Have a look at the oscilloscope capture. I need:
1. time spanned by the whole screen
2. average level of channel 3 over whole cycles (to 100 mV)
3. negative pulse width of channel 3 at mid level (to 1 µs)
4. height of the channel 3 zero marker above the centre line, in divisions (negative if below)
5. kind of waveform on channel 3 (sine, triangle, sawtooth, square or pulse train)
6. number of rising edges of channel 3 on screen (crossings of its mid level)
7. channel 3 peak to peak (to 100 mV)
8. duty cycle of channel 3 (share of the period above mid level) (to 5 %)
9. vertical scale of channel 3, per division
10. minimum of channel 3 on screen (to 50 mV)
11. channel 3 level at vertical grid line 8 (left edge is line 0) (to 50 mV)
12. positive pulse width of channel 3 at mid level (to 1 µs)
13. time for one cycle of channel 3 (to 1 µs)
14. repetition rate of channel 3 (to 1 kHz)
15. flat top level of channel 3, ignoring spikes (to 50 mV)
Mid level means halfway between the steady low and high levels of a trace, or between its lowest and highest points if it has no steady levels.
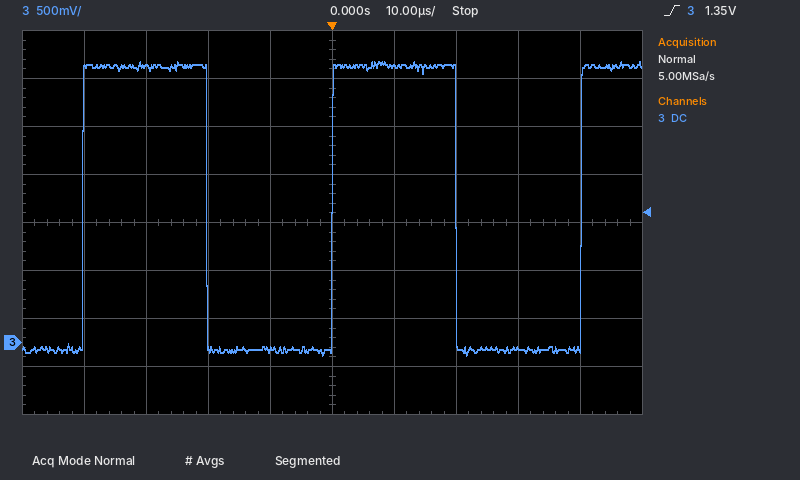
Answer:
100 µs
1.4 V
20 µs
-2.5 div
square
3
3.10 V
50 %
500 mV
-150 mV
-50 mV
20 µs
40 µs
25 kHz
2.90 V
